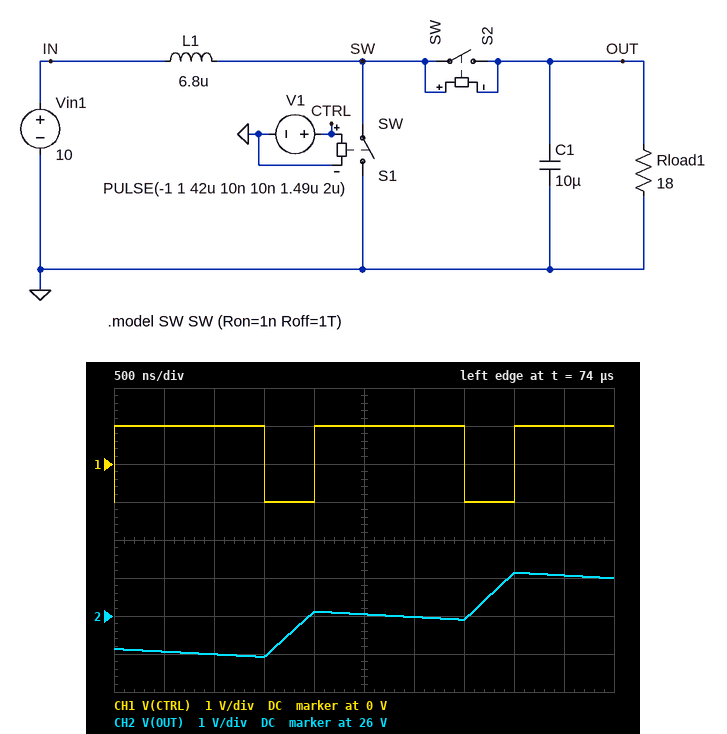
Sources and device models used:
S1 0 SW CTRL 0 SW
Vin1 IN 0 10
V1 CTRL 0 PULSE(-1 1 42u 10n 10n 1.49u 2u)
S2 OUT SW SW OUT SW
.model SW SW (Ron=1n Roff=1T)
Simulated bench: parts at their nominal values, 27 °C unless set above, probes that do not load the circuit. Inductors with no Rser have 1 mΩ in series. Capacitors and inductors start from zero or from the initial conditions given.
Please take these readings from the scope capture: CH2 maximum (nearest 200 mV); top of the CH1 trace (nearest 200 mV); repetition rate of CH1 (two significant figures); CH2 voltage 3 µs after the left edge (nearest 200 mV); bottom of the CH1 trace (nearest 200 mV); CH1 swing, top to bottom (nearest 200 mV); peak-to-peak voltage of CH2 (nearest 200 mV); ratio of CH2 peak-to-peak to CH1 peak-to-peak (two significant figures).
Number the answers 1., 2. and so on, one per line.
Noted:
1. 27.2 V
2. 1.0 V
3. 500 kHz
4. 26.0 V
5. -1.0 V
6. 2.0 V
7. 2.2 V
8. 1.1
